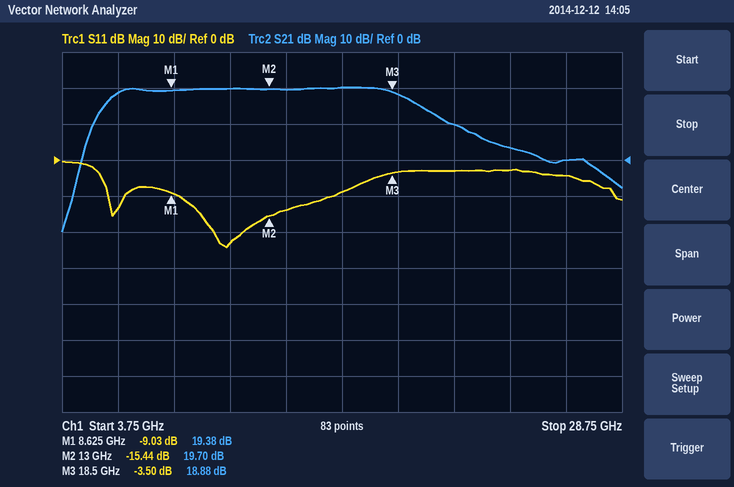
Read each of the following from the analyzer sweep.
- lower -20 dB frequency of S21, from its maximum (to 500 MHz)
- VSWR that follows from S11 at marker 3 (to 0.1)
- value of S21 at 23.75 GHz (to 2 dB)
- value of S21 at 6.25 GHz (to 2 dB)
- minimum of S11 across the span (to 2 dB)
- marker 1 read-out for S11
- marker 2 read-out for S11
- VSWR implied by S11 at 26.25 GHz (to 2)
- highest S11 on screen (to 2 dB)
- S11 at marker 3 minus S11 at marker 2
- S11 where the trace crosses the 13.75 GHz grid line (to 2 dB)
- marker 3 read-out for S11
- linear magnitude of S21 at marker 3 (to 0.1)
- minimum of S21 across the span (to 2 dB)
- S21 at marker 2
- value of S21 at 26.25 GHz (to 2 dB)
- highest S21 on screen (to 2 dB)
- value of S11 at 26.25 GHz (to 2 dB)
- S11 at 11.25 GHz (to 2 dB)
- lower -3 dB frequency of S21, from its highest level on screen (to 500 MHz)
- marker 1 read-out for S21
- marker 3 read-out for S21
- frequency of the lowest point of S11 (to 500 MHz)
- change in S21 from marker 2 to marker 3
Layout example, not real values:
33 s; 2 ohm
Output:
4.5 GHz; 5.0; 4 dB; 18 dB; -24 dB; -9.03 dB; -15.44 dB; 4; 0 dB; 11.94 dB; -14 dB; -3.50 dB; 8.8; -20 dB; 19.70 dB; 0 dB; 20 dB; -4 dB; -24 dB; 6.0 GHz; 19.38 dB; 18.88 dB; 11.0 GHz; -0.82 dB
